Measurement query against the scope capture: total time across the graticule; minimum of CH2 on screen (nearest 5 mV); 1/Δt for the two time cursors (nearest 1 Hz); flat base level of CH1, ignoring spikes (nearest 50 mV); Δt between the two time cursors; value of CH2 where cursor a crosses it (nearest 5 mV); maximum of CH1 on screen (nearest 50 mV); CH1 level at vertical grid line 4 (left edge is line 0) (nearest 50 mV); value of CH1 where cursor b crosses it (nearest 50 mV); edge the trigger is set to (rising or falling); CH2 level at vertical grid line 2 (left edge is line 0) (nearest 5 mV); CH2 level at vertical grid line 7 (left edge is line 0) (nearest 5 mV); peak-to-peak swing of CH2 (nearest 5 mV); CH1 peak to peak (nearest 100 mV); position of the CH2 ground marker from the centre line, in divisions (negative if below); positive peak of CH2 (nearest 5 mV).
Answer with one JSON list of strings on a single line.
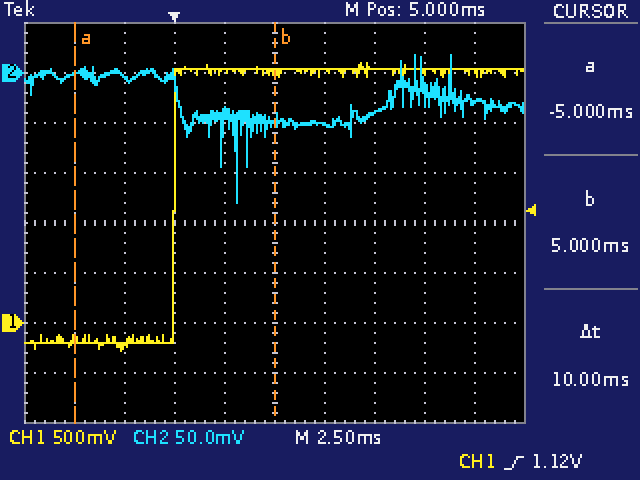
["25 ms", "-130 mV", "100 Hz", "-200 mV", "10 ms", "0 mV", "2.60 V", "2.50 V", "2.50 V", "rising", "-5 mV", "-40 mV", "150 mV", "2.90 V", "+3.0 div", "20 mV"]
